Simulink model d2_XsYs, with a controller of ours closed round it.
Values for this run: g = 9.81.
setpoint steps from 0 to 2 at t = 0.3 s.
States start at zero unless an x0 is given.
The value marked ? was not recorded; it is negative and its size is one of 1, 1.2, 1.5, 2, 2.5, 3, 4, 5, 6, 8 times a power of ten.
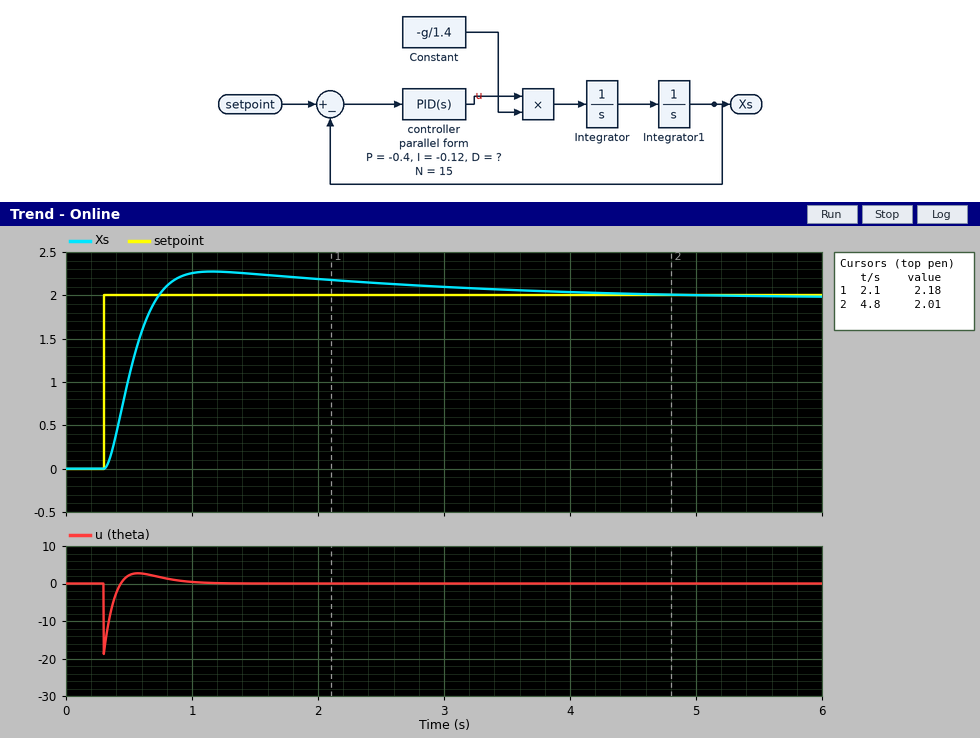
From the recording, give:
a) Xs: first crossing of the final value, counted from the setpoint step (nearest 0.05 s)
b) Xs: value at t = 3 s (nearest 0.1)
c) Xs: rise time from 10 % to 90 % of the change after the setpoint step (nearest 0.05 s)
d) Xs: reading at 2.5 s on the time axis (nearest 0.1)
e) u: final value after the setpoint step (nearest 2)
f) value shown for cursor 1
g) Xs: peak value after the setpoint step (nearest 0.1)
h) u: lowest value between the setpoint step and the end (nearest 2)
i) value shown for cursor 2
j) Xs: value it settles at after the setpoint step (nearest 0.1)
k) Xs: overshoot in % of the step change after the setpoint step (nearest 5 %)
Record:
0.45 s
2.1
0.30 s
2.1
0
2.18
2.3
-18
2.01
2.0
15 %
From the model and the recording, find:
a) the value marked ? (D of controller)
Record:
-0.6
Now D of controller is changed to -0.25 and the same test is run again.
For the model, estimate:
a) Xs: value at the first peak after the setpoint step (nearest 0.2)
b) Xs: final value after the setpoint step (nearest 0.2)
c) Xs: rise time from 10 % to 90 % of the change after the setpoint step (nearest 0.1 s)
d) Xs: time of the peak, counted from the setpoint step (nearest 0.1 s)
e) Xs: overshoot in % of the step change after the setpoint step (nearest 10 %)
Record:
2.8
2.0
0.5 s
1.4 s
40 %
